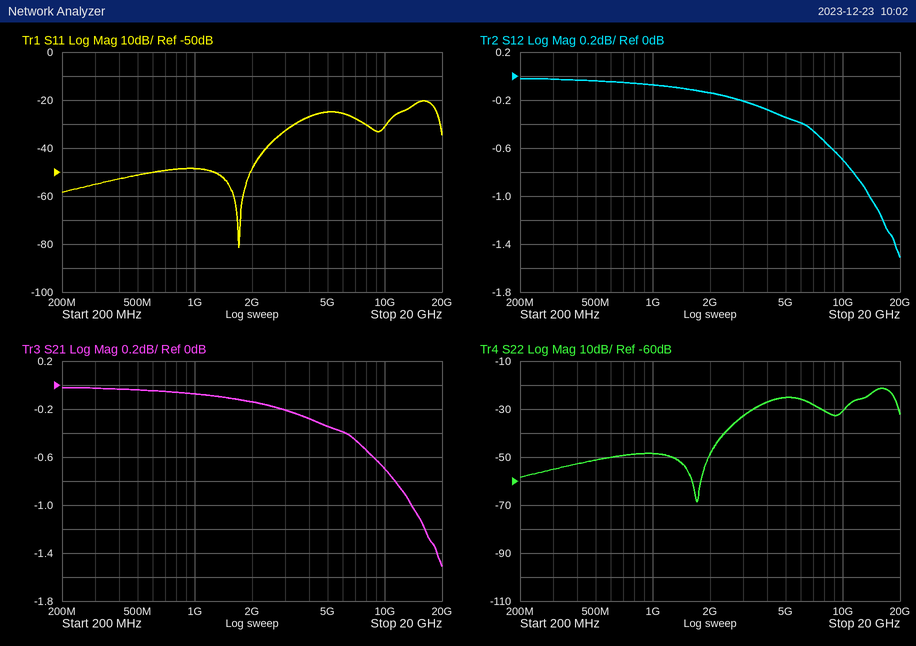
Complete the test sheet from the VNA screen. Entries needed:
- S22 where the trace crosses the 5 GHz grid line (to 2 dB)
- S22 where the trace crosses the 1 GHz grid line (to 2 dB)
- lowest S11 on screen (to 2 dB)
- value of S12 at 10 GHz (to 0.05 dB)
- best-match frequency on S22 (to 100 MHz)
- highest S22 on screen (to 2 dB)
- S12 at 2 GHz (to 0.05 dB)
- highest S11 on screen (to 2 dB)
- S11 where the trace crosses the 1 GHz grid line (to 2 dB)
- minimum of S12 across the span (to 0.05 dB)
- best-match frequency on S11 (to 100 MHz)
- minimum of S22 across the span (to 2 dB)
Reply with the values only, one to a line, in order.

-26 dB
-48 dB
-82 dB
-0.70 dB
1.7 GHz
-22 dB
-0.15 dB
-20 dB
-48 dB
-1.50 dB
1.7 GHz
-68 dB
